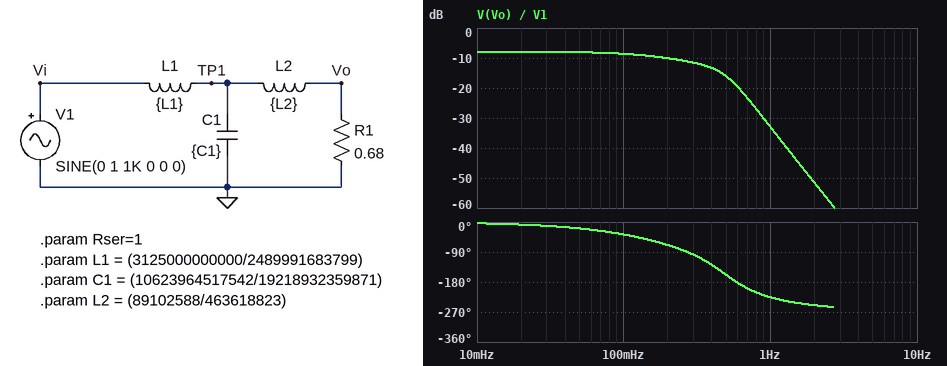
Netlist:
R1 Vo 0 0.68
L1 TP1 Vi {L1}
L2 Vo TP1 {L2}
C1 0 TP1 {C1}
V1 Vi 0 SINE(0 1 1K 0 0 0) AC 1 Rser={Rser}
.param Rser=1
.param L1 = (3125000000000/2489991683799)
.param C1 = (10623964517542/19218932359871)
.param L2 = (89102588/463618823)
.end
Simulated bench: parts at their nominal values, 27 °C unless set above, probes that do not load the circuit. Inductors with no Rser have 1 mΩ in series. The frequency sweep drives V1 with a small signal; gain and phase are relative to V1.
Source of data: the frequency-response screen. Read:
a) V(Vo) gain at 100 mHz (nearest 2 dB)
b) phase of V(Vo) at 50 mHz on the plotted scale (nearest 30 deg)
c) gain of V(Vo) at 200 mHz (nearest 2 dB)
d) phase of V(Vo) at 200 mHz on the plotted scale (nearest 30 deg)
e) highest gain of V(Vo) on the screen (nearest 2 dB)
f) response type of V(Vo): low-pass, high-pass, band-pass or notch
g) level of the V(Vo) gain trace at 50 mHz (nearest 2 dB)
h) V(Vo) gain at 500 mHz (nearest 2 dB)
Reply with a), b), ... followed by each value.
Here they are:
a) -8 dB
b) -30 deg
c) -10 dB
d) -60 deg
e) -8 dB
f) low-pass
g) -8 dB
h) -16 dB
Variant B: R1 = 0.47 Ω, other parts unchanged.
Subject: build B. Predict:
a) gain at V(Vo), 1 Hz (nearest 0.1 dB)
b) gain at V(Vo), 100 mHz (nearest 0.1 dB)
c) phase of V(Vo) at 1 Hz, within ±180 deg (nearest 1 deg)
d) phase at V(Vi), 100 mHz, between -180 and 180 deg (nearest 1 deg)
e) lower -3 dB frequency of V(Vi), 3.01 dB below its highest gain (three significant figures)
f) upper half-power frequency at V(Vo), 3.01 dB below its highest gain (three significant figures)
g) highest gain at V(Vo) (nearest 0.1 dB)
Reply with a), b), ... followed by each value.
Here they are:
a) -35.3 dB
b) -11.0 dB
c) 125 deg
d) 30 deg
e) 163 mHz
f) 212 mHz
g) -9.9 dB
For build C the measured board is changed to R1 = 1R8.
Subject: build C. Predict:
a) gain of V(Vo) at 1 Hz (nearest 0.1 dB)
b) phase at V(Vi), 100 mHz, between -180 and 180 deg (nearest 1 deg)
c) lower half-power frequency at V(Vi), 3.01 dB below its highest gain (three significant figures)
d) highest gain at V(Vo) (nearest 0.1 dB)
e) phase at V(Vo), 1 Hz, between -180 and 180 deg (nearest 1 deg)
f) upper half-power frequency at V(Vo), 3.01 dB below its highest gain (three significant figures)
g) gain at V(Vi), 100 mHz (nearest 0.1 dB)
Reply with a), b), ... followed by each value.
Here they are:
a) -29.5 dB
b) 0 deg
c) 275 mHz
d) -3.5 dB
e) 161 deg
f) 279 mHz
g) -4.7 dB
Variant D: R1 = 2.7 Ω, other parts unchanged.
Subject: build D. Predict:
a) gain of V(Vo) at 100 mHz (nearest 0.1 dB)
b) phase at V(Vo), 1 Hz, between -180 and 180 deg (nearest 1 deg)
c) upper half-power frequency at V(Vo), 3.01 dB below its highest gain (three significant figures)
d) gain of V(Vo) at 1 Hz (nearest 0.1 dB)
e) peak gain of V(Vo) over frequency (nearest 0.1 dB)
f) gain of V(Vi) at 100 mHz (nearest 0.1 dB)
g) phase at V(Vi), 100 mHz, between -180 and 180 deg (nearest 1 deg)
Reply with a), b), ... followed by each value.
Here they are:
a) -2.1 dB
b) 169 deg
c) 266 mHz
d) -29.0 dB
e) -1.7 dB
f) -4.1 dB
g) -8 deg
